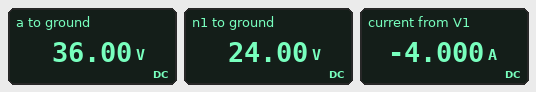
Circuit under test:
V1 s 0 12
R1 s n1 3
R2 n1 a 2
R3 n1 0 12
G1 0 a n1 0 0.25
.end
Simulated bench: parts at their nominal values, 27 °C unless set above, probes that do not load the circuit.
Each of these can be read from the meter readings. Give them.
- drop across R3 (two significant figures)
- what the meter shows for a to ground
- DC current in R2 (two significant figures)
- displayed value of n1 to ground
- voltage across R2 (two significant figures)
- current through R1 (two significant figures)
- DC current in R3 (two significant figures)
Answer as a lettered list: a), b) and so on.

a) 24 V
b) 36.00 V
c) 6.0 A
d) 24.00 V
e) 12 V
f) 4.0 A
g) 2.0 A
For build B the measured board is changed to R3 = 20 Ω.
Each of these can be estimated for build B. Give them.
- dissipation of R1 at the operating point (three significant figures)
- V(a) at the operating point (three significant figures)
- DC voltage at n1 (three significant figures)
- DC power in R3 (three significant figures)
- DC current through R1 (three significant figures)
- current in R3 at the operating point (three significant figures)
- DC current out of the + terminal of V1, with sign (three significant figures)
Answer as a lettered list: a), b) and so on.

a) 108 W
b) 45.0 V
c) 30.0 V
d) 45.0 W
e) 6.00 A
f) 1.50 A
g) -6.00 A
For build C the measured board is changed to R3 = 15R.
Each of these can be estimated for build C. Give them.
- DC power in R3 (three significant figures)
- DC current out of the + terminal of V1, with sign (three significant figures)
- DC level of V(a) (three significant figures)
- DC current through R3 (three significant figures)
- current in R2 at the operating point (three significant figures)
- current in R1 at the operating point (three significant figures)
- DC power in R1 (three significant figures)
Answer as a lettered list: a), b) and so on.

a) 47.4 W
b) -4.89 A
c) 40.0 V
d) 1.78 A
e) 6.67 A
f) 4.89 A
g) 71.7 W
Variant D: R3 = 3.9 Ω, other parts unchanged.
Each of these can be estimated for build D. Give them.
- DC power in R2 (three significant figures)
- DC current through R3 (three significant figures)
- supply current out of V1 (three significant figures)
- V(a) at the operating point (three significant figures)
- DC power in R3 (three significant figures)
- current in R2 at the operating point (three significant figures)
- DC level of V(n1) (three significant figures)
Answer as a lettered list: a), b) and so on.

a) 17.3 W
b) 3.02 A
c) 75.5 mA
d) 17.7 V
e) 35.5 W
f) 2.94 A
g) 11.8 V
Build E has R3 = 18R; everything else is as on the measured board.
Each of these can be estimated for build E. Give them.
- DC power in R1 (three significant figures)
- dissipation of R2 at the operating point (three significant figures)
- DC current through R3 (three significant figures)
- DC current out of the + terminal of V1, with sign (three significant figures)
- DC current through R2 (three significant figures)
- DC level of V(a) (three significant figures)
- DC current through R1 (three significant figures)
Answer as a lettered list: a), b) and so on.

a) 94.1 W
b) 104 W
c) 1.60 A
d) -5.60 A
e) 7.20 A
f) 43.2 V
g) 5.60 A
